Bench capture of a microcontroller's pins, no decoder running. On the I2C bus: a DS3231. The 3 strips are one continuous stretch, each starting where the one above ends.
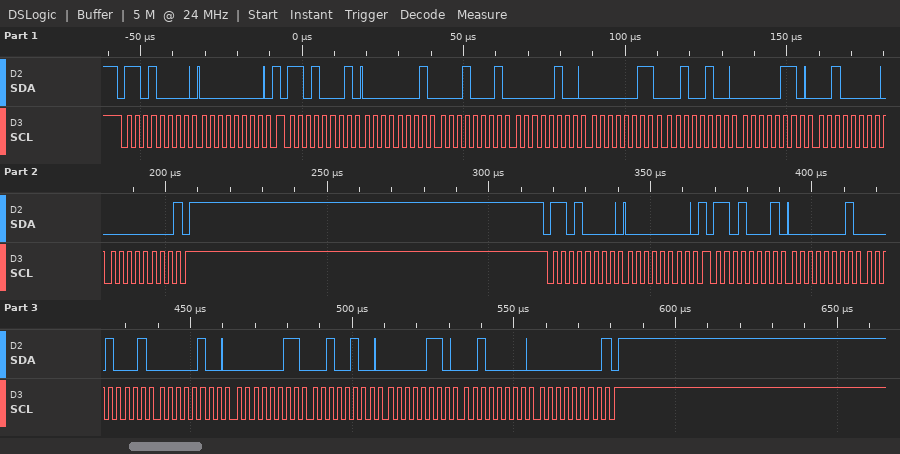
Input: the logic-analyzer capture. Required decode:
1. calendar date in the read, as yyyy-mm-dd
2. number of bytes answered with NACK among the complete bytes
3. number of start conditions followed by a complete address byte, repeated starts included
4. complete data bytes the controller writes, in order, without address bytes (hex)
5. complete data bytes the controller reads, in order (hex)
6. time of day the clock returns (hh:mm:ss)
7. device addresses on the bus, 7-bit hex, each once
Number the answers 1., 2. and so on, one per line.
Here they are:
1. 2020-06-24
2. 2
3. 4
4. 00 00
5. 01 11 04 03 24 06 20 00 01 11 04 03 24 06 20 00
6. 04:11:01
7. 0x68
